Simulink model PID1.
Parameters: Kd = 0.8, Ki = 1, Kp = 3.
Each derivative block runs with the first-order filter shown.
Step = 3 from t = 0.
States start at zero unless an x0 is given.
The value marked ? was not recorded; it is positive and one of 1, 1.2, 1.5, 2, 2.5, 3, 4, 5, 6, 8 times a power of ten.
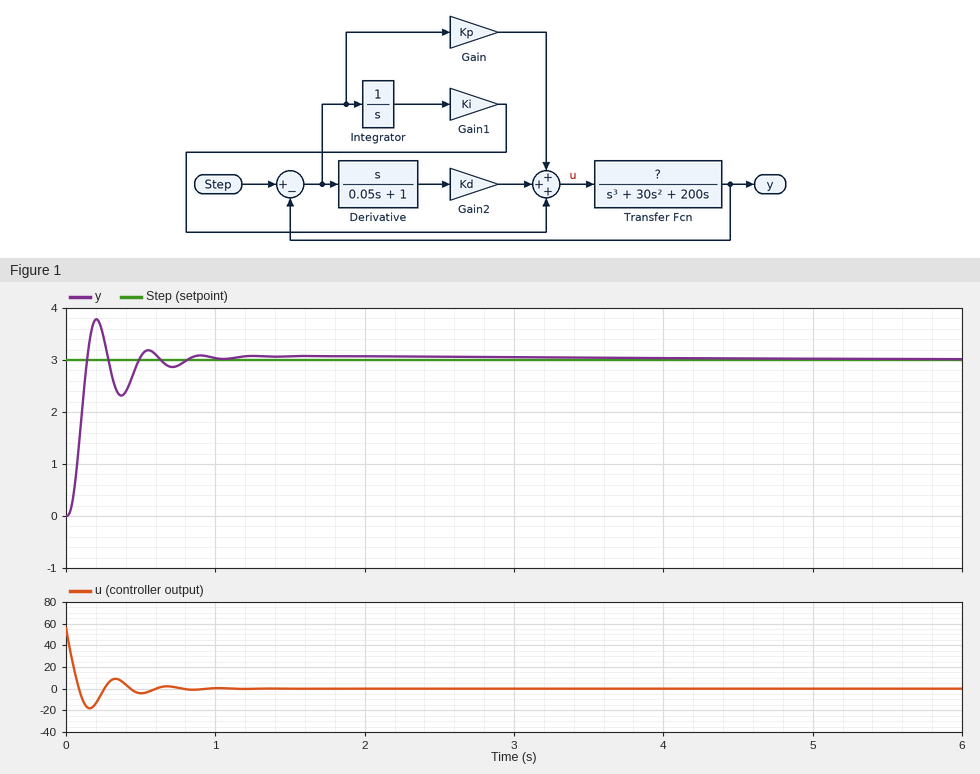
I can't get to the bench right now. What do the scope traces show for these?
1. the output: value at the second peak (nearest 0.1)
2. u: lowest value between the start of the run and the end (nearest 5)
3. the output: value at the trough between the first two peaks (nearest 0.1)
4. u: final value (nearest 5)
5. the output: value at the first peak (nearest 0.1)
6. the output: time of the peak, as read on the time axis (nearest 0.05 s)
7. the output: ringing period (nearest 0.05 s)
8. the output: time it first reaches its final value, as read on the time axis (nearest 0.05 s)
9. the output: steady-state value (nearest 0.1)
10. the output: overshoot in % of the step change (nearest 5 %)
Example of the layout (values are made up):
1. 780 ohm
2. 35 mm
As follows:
1. 3.2
2. -20
3. 2.3
4. 0
5. 3.8
6. 0.20 s
7. 0.35 s
8. 0.15 s
9. 3.0
10. 25 %
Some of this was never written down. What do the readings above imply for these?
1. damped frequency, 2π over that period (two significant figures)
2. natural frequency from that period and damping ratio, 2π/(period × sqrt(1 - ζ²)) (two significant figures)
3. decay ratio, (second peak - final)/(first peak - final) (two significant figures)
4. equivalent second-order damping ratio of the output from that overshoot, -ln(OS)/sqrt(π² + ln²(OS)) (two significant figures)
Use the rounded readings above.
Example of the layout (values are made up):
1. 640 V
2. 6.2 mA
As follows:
1. 18 rad/s
2. 20 rad/s
3. 0.25
4. 0.40
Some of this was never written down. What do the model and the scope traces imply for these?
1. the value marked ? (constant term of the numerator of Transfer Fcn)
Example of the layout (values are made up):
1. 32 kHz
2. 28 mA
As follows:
1. 600
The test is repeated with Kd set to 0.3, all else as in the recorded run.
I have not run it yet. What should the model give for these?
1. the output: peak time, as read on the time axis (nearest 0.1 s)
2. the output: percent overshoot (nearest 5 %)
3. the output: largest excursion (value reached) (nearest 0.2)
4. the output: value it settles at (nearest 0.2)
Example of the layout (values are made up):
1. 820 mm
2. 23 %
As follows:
1. 0.3 s
2. 20 %
3. 3.6
4. 3.0
